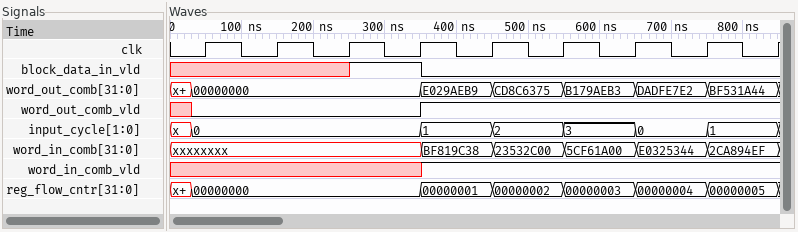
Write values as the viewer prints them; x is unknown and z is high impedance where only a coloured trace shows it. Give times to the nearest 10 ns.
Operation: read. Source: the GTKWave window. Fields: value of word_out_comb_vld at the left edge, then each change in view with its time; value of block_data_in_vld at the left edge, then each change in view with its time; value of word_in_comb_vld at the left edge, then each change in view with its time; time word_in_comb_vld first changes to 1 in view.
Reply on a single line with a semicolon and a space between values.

x, 0 at 30 ns, 1 at 350 ns; x, 1 at 250 ns, 0 at 350 ns; x, 1 at 350 ns; 350 ns
